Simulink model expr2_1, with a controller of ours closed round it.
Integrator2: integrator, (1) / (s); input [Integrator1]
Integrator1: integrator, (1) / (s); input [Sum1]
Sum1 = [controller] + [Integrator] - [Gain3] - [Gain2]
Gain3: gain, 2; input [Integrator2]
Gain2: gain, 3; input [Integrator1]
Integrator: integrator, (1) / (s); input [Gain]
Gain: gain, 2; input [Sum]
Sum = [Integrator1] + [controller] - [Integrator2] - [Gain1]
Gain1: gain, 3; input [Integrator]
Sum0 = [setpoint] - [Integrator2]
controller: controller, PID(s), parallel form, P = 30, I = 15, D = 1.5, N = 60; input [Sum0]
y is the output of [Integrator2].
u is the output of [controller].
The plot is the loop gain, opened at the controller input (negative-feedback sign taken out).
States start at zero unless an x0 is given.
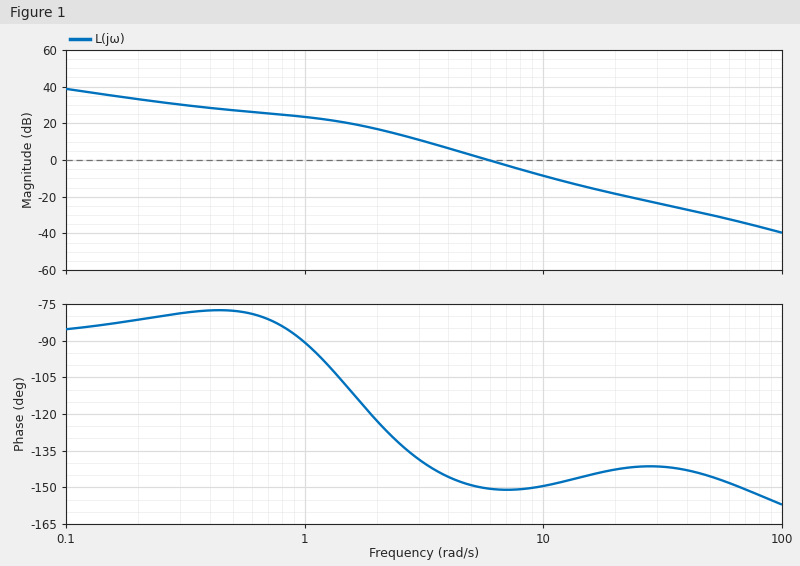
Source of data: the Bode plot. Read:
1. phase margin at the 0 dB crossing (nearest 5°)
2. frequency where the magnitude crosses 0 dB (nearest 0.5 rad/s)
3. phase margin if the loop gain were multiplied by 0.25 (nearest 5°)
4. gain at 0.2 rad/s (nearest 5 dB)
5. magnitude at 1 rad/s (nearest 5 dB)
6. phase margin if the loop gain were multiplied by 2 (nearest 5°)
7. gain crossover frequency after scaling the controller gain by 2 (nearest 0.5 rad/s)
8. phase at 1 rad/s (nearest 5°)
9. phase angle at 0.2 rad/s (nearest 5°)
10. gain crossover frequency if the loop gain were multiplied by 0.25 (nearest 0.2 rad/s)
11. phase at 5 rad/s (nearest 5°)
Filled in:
30°
6.0 rad/s
45°
35 dB
25 dB
30°
8.5 rad/s
-90°
-80°
2.8 rad/s
-150°
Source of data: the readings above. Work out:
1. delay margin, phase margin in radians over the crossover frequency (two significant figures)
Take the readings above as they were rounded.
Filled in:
0.087 s
